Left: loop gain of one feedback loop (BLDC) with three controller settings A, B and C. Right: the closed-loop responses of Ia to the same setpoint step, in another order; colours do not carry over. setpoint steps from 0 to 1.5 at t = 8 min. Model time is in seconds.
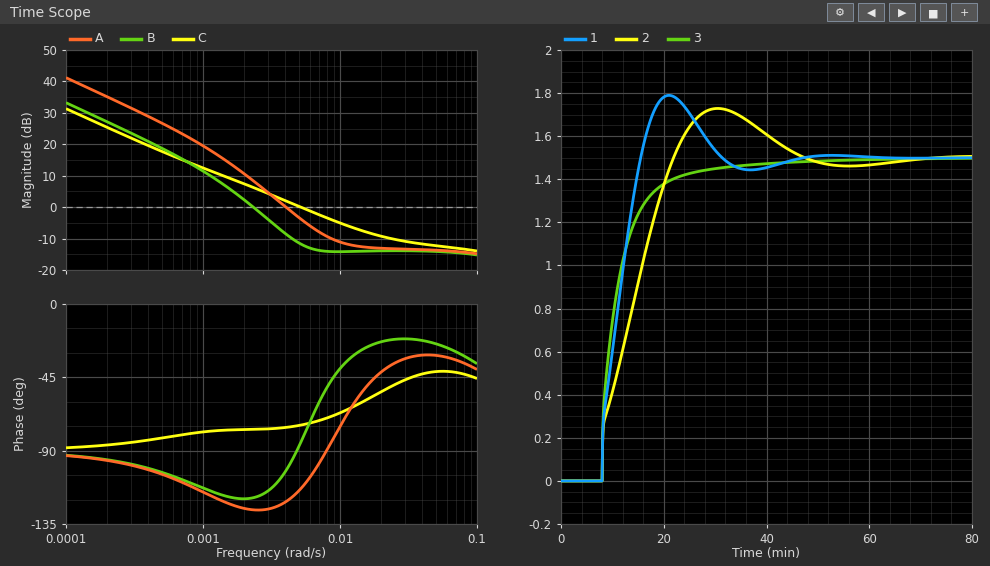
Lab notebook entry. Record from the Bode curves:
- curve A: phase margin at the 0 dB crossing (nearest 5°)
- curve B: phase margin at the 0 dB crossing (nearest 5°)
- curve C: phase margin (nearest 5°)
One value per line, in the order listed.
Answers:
60°
60°
105°
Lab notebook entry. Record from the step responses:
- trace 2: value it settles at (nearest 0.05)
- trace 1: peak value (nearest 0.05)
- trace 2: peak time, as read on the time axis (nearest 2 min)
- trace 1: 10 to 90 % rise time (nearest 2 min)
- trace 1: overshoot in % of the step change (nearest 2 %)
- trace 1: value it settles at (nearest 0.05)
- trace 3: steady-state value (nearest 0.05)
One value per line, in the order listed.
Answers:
1.50
1.80
30 min
6 min
20 %
1.50
1.50
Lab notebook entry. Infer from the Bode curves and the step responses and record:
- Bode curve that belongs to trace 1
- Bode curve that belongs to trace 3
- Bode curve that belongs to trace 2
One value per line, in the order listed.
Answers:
A
C
B
